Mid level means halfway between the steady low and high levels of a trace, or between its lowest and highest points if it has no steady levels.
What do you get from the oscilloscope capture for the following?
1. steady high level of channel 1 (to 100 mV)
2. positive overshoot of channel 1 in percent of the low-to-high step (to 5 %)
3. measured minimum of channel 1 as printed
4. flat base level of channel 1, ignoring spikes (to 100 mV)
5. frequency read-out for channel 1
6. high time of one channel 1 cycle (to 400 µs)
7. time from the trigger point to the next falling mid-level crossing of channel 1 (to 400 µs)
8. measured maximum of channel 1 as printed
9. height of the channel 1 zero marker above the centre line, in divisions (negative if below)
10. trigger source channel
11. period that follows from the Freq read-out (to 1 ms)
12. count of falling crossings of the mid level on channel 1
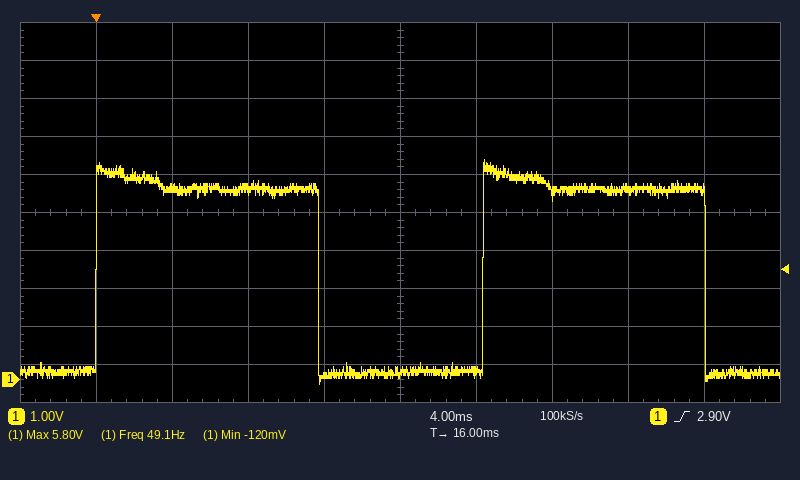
5.0 V
15 %
-120 mV
200 mV
49.1 Hz
11.6 ms
11.6 ms
5.80 V
-4.4 div
channel 1
20 ms
2
